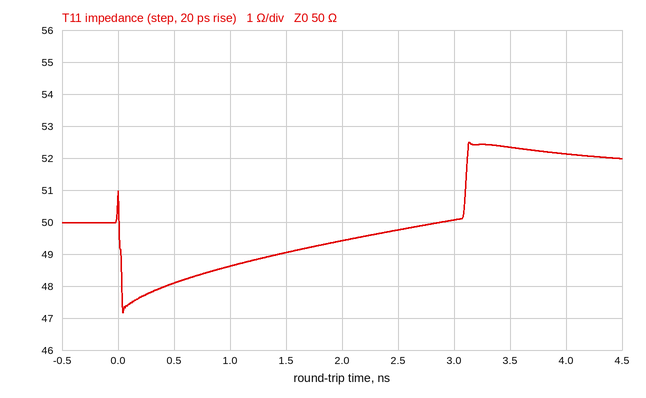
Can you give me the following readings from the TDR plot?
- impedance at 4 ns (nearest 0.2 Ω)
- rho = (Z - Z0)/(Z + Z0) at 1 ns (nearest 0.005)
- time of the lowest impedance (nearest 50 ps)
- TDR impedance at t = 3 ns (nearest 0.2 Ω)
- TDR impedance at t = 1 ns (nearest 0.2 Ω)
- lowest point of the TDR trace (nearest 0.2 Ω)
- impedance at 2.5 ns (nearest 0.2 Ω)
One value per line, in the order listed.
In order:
52.2 Ω
-0.015
50 ps
50.0 Ω
48.6 Ω
47.2 Ω
49.8 Ω
